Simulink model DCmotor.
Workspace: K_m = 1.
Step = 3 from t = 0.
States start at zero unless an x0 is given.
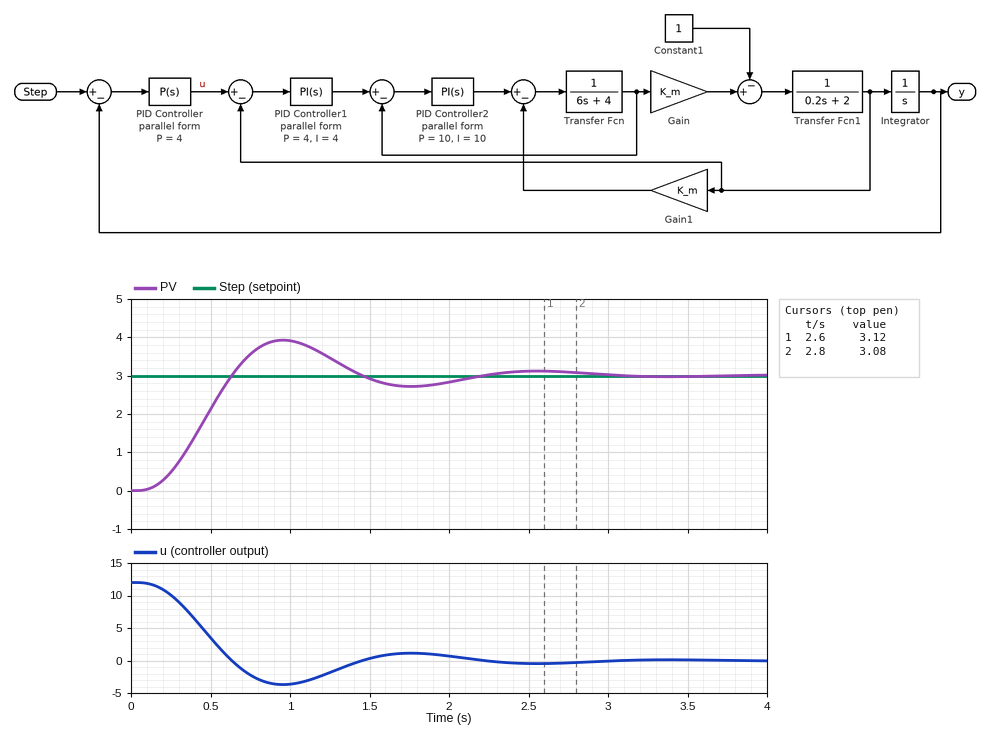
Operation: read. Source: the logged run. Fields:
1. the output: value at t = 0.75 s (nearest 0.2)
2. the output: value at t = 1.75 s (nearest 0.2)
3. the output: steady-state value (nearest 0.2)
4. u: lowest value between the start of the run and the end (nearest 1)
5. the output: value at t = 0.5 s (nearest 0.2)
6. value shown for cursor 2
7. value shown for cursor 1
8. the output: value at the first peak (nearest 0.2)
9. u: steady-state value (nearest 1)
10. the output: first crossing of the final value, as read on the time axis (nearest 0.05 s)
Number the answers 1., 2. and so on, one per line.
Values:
1. 3.6
2. 2.8
3. 3.0
4. -4
5. 2.2
6. 3.08
7. 3.12
8. 4.0
9. 0
10. 0.65 s
